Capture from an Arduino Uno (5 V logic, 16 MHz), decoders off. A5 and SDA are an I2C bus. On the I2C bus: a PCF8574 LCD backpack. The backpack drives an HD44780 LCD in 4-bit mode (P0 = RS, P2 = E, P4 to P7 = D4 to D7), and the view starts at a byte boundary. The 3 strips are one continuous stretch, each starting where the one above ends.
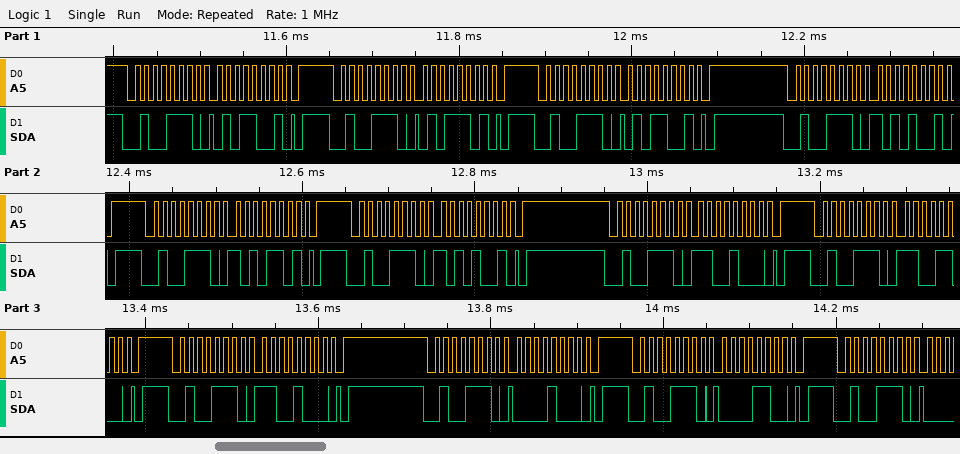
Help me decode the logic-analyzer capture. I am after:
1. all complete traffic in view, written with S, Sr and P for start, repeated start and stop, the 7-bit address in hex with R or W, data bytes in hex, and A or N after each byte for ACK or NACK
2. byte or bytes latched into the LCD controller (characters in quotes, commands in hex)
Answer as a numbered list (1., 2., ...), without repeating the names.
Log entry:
1. S 27W A 59 A P S 27W A 5D A P S 27W A 59 A P S 27W A A9 A P S 27W A AD A P S 27W A A9 A P S 27W A C8 A P S 27W A CC A P S 27W A C8 A P S 27W A 08 A P S 27W A 0C A P S 27W A
2. 'Z'
